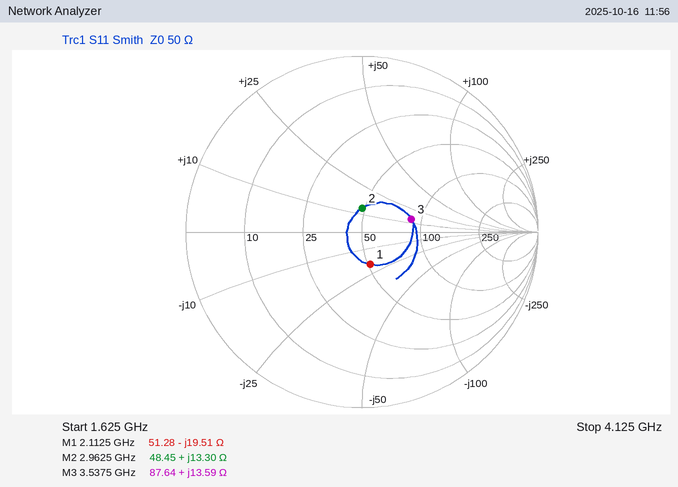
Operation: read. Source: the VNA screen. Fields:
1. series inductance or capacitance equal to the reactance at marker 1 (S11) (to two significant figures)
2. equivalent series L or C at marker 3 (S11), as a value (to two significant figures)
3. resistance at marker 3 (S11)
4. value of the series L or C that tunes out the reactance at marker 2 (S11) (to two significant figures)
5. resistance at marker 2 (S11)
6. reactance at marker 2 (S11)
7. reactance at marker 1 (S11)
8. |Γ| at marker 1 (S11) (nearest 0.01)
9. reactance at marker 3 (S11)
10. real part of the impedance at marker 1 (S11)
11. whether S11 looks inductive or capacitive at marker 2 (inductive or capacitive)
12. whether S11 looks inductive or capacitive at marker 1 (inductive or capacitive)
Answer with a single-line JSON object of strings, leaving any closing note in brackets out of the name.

{"series inductance or capacitance equal to the reactance at marker 1 (S11)": "3.9 pF", "equivalent series L or C at marker 3 (S11), as a value": "610 pH", "resistance at marker 3": "87.64 Ω", "value of the series L or C that tunes out the reactance at marker 2 (S11)": "4.0 pF", "resistance at marker 2": "48.45 Ω", "reactance at marker 2": "+13.30 Ω", "reactance at marker 1": "-19.51 Ω", "|Γ| at marker 1 (S11)": "0.19", "reactance at marker 3": "+13.59 Ω", "real part of the impedance at marker 1": "51.28 Ω", "whether S11 looks inductive or capacitive at marker 2": "inductive", "whether S11 looks inductive or capacitive at marker 1": "capacitive"}
